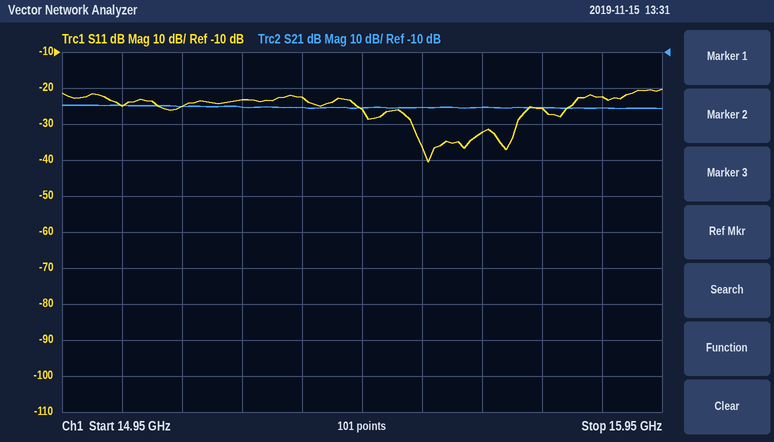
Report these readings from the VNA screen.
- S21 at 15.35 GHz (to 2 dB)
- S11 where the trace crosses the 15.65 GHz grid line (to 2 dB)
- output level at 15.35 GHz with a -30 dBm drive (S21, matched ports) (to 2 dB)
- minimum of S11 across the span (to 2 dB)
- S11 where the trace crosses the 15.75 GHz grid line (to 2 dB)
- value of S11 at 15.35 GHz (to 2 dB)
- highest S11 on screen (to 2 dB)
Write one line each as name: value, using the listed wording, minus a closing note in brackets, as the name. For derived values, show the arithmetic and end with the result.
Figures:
S21 at 15.35 GHz: -26 dB
S11 where the trace crosses the 15.65 GHz grid line: -32 dB
output level at 15.35 GHz with a -30 dBm drive (S21, matched ports): -30 dBm + (-26 dB) = -56 dBm
minimum of S11 across the span: -40 dB
S11 where the trace crosses the 15.75 GHz grid line: -26 dB
value of S11 at 15.35 GHz: -22 dB
highest S11 on screen: -20 dB
